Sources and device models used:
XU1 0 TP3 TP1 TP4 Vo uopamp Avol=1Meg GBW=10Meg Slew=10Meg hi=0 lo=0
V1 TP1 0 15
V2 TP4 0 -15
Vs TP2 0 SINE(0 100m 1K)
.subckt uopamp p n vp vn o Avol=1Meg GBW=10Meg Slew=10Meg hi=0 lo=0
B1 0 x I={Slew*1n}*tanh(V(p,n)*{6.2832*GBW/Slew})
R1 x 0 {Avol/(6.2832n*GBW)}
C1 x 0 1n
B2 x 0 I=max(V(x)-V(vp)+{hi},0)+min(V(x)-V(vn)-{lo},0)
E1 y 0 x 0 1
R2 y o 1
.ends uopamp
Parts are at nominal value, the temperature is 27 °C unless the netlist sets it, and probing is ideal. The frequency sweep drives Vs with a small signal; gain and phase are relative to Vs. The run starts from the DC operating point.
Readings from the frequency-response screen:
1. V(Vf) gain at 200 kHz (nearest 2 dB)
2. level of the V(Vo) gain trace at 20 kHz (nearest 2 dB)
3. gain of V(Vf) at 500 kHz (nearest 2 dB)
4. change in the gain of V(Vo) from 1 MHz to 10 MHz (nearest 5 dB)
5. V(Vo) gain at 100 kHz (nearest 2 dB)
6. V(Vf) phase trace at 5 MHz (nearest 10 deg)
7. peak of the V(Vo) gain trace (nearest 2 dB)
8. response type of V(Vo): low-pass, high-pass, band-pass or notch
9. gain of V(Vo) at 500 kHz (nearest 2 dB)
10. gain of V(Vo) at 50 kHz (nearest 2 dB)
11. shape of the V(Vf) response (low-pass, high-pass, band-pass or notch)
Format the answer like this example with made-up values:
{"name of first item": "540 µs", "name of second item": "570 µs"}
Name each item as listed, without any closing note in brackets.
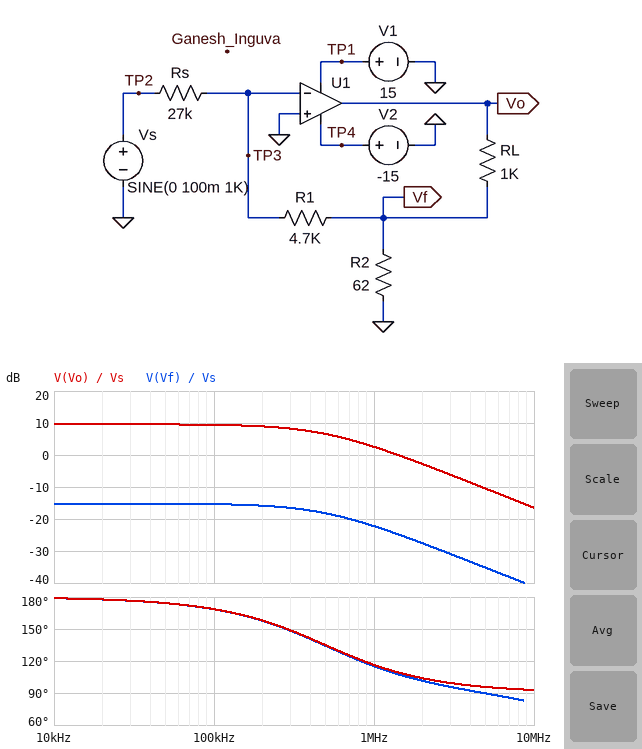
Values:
{"V(Vf) gain at 200 kHz": "-16 dB", "level of the V(Vo) gain trace at 20 kHz": "10 dB", "gain of V(Vf) at 500 kHz": "-18 dB", "change in the gain of V(Vo) from 1 MHz to 10 MHz": "-20 dB", "V(Vo) gain at 100 kHz": "10 dB", "V(Vf) phase trace at 5 MHz": "90 deg", "peak of the V(Vo) gain trace": "10 dB", "response type of V(Vo): low-pass, high-pass, band-pass or notch": "low-pass", "gain of V(Vo) at 500 kHz": "6 dB", "gain of V(Vo) at 50 kHz": "10 dB", "shape of the V(Vf) response": "low-pass"}
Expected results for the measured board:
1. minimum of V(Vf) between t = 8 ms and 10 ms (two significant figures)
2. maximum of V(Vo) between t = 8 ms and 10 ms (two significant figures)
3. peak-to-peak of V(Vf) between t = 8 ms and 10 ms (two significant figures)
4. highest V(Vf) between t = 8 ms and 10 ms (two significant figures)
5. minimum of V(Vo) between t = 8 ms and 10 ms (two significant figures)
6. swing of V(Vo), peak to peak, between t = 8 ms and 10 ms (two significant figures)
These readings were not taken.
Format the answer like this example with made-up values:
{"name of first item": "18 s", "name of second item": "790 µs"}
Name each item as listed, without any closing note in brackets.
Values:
{"minimum of V(Vf) between t = 8 ms and 10 ms": "-17 mV", "maximum of V(Vo) between t = 8 ms and 10 ms": "300 mV", "peak-to-peak of V(Vf) between t = 8 ms and 10 ms": "35 mV", "highest V(Vf) between t = 8 ms and 10 ms": "17 mV", "minimum of V(Vo) between t = 8 ms and 10 ms": "-300 mV", "swing of V(Vo), peak to peak, between t = 8 ms and 10 ms": "600 mV"}
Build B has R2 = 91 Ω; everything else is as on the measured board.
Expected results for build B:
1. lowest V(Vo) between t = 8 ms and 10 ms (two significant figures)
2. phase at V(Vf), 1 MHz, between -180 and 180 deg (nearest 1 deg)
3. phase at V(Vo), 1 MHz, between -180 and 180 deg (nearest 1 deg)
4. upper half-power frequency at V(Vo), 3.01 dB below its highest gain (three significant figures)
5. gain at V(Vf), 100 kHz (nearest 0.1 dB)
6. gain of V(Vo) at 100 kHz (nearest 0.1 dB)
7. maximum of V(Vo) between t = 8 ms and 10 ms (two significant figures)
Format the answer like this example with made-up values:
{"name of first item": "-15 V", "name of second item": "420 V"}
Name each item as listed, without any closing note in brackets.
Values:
{"lowest V(Vo) between t = 8 ms and 10 ms": "-210 mV", "phase at V(Vf), 1 MHz, between -180 and 180 deg": "124 deg", "phase at V(Vo), 1 MHz, between -180 and 180 deg": "125 deg", "upper half-power frequency at V(Vo), 3.01 dB below its highest gain": "708 kHz", "gain at V(Vf), 100 kHz": "-15.3 dB", "gain of V(Vo) at 100 kHz": "6.5 dB", "maximum of V(Vo) between t = 8 ms and 10 ms": "210 mV"}
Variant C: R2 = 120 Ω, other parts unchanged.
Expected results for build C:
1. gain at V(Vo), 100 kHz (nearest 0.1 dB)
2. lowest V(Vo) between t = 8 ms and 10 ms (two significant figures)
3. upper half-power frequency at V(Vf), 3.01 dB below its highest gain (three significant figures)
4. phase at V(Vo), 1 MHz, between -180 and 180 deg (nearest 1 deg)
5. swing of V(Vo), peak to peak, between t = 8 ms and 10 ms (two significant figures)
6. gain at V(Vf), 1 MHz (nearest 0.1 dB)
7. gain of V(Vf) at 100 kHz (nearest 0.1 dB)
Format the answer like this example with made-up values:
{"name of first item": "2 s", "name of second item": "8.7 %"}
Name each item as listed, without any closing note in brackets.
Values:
{"gain at V(Vo), 100 kHz": "4.4 dB", "lowest V(Vo) between t = 8 ms and 10 ms": "-170 mV", "upper half-power frequency at V(Vf), 3.01 dB below its highest gain": "909 kHz", "phase at V(Vo), 1 MHz, between -180 and 180 deg": "132 deg", "swing of V(Vo), peak to peak, between t = 8 ms and 10 ms": "330 mV", "gain at V(Vf), 1 MHz": "-18.6 dB", "gain of V(Vf) at 100 kHz": "-15.2 dB"}
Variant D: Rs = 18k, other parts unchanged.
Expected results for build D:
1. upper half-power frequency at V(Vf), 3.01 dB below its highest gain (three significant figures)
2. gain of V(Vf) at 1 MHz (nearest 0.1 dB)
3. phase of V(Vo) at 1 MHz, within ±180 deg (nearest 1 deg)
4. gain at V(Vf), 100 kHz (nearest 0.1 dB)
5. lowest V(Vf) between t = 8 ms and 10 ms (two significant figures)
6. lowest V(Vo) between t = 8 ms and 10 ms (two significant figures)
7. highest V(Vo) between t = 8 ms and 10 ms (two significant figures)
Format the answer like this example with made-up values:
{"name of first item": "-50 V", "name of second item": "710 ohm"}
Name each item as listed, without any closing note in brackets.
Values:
{"upper half-power frequency at V(Vf), 3.01 dB below its highest gain": "461 kHz", "gain of V(Vf) at 1 MHz": "-19.2 dB", "phase of V(Vo) at 1 MHz, within ±180 deg": "115 deg", "gain at V(Vf), 100 kHz": "-11.9 dB", "lowest V(Vf) between t = 8 ms and 10 ms": "-26 mV", "lowest V(Vo) between t = 8 ms and 10 ms": "-450 mV", "highest V(Vo) between t = 8 ms and 10 ms": "450 mV"}
